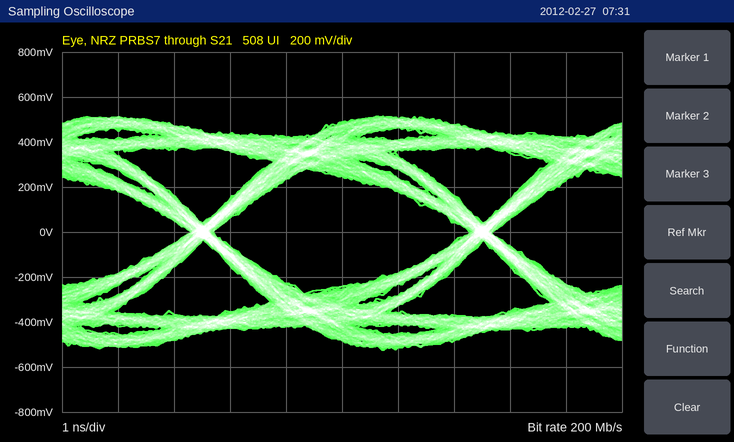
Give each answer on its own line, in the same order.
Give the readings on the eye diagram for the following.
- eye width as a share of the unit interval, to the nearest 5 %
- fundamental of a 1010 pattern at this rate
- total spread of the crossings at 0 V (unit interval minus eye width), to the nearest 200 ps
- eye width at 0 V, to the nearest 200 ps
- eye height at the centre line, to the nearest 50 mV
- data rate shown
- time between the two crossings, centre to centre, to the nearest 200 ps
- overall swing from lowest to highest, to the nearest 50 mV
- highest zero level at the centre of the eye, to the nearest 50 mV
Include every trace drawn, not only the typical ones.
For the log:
90 %
100 MHz
400 ps
4.6 ns
500 mV
200 Mb/s
5.0 ns
1.05 V
-250 mV
